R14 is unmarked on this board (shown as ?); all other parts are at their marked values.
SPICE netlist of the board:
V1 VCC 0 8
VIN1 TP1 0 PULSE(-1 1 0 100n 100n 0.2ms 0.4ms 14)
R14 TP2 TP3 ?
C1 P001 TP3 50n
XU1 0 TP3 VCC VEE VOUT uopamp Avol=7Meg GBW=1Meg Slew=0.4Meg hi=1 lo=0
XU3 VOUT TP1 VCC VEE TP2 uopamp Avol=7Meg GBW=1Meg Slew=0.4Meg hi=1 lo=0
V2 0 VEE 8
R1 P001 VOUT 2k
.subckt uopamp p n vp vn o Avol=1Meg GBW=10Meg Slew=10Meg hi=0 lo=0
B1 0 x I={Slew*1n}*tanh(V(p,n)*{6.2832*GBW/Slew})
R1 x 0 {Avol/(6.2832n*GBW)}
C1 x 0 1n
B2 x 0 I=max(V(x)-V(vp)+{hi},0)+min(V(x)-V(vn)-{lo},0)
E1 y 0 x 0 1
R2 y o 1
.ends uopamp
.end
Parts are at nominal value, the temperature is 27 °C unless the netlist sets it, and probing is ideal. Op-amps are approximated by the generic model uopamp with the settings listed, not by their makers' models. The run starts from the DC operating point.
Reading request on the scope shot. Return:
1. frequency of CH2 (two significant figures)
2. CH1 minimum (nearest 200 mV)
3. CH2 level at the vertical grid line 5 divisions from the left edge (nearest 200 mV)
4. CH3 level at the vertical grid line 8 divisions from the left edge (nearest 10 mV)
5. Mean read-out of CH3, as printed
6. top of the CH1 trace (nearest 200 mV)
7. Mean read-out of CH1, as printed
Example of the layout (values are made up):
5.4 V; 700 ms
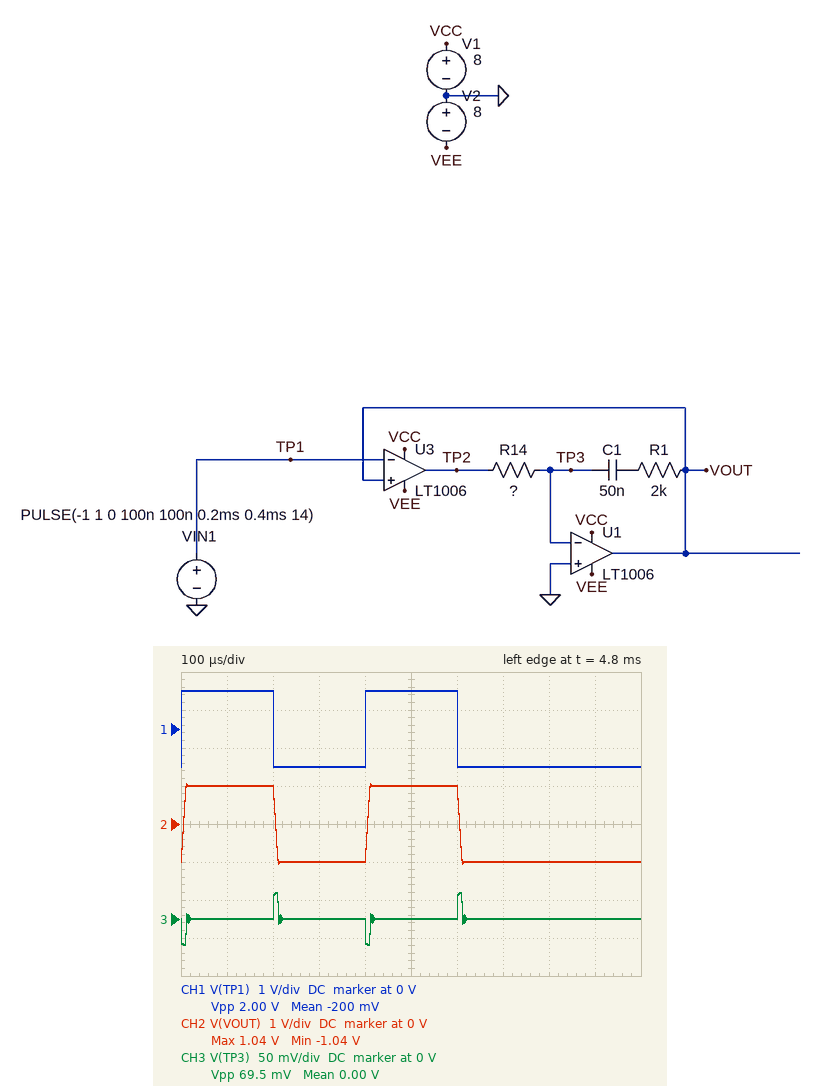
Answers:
2.5 kHz; -1.0 V; 1.0 V; 0 V; 0.00 V; 1.0 V; -200 mV
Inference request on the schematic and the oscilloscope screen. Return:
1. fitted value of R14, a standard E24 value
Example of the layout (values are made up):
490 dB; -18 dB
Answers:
4.3 kΩ
